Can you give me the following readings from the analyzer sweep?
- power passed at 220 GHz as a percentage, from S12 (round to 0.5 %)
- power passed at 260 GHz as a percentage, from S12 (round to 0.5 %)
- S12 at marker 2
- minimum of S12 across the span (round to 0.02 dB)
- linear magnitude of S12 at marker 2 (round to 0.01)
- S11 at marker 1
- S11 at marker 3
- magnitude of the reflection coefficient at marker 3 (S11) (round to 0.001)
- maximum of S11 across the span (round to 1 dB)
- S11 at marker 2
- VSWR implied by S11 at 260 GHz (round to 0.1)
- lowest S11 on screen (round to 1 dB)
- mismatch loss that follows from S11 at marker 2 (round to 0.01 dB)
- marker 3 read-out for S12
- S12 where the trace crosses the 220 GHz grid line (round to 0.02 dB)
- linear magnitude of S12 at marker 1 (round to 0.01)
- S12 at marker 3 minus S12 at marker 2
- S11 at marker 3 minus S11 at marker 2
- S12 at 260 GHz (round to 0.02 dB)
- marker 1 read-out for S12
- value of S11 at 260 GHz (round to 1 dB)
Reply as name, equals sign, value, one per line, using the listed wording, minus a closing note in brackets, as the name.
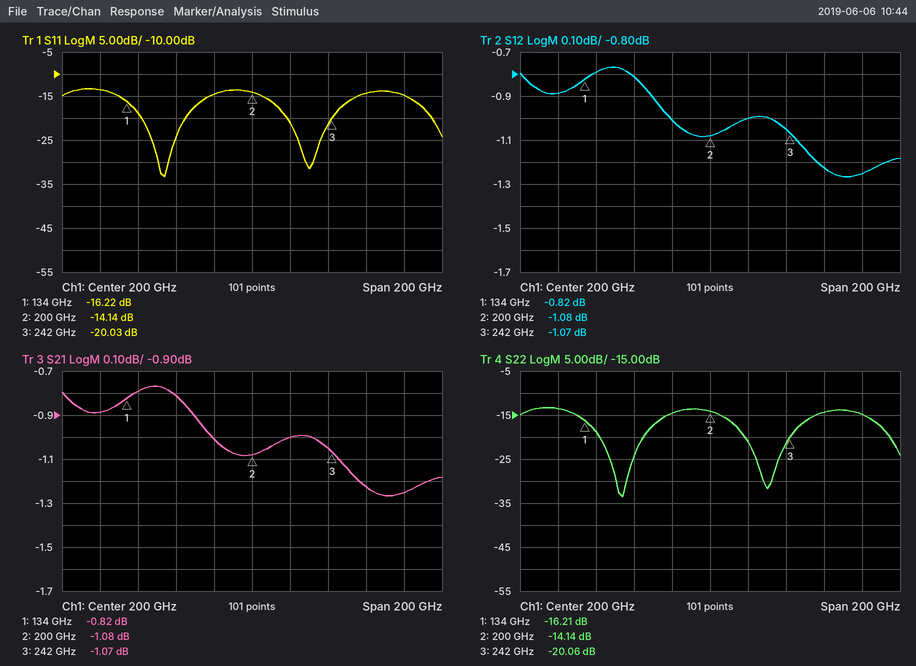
power passed at 220 GHz as a percentage, from S12 = 79.5 %
power passed at 260 GHz as a percentage, from S12 = 75.5 %
S12 at marker 2 = -1.08 dB
minimum of S12 across the span = -1.26 dB
linear magnitude of S12 at marker 2 = 0.88
S11 at marker 1 = -16.22 dB
S11 at marker 3 = -20.03 dB
magnitude of the reflection coefficient at marker 3 (S11) = 0.100
maximum of S11 across the span = -13 dB
S11 at marker 2 = -14.14 dB
VSWR implied by S11 at 260 GHz = 1.5
lowest S11 on screen = -33 dB
mismatch loss that follows from S11 at marker 2 = 0.17 dB
marker 3 read-out for S12 = -1.07 dB
S12 where the trace crosses the 220 GHz grid line = -1.00 dB
linear magnitude of S12 at marker 1 = 0.91
S12 at marker 3 minus S12 at marker 2 = 0.01 dB
S11 at marker 3 minus S11 at marker 2 = -5.89 dB
S12 at 260 GHz = -1.22 dB
marker 1 read-out for S12 = -0.82 dB
value of S11 at 260 GHz = -14 dB
